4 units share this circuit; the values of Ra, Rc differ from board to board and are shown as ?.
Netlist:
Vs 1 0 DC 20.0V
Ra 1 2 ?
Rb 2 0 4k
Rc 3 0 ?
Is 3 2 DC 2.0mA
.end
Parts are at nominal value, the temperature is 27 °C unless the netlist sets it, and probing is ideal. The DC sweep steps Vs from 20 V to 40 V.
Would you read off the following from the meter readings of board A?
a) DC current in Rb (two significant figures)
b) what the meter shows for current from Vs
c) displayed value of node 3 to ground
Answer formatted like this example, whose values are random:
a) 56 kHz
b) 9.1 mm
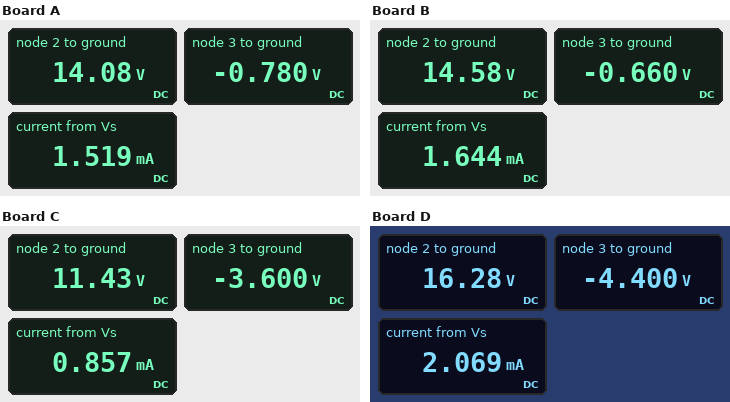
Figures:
a) 3.5 mA
b) 1.519 mA
c) -0.780 V
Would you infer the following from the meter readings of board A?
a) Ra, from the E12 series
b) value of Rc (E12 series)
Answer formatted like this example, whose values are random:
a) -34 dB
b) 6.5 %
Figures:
a) 3.9 kΩ
b) 390 Ω
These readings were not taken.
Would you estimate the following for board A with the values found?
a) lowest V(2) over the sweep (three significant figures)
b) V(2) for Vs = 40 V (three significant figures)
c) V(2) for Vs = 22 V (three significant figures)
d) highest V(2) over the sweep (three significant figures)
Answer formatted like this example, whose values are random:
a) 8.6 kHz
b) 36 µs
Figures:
a) 14.1 V
b) 24.2 V
c) 15.1 V
d) 24.2 V
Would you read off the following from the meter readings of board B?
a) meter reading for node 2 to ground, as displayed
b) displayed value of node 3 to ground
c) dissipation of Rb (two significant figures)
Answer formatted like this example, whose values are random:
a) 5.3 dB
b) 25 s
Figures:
a) 14.58 V
b) -0.660 V
c) 53 mW
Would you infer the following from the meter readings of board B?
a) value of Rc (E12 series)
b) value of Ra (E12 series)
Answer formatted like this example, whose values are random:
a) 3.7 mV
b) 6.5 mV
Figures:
a) 330 Ω
b) 3.3 kΩ
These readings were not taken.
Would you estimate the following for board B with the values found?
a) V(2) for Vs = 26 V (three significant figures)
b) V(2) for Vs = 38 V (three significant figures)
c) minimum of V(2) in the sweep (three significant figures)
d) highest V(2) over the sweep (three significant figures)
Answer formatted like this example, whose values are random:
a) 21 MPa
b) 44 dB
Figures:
a) 17.9 V
b) 24.4 V
c) 14.6 V
d) 25.5 V
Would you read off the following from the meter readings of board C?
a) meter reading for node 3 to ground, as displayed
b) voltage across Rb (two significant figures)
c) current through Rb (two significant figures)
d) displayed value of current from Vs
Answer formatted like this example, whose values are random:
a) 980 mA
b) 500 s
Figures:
a) -3.600 V
b) 11 V
c) 2.9 mA
d) 0.857 mA
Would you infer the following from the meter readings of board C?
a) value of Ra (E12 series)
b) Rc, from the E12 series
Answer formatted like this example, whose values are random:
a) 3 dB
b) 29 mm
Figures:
a) 10 kΩ
b) 1.8 kΩ
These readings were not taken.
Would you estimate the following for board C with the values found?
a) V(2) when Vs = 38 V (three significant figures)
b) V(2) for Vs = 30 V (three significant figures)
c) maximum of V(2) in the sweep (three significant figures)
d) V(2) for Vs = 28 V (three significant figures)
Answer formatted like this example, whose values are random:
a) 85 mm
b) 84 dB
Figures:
a) 16.6 V
b) 14.3 V
c) 17.1 V
d) 13.7 V
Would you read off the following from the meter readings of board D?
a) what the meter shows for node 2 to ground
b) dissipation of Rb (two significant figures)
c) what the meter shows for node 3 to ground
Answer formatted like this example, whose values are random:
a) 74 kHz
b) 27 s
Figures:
a) 16.28 V
b) 66 mW
c) -4.400 V
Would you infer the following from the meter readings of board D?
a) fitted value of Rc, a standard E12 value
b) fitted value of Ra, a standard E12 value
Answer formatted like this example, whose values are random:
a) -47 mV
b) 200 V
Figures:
a) 2.2 kΩ
b) 1.8 kΩ
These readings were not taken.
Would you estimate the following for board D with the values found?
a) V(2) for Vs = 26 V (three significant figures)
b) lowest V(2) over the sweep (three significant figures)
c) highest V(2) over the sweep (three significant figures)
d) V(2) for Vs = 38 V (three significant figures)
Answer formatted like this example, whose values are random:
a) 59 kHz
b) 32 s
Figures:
a) 20.4 V
b) 16.3 V
c) 30.1 V
d) 28.7 V
